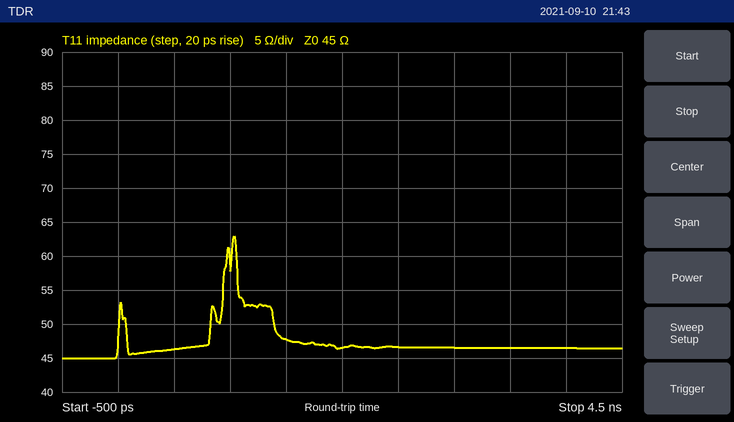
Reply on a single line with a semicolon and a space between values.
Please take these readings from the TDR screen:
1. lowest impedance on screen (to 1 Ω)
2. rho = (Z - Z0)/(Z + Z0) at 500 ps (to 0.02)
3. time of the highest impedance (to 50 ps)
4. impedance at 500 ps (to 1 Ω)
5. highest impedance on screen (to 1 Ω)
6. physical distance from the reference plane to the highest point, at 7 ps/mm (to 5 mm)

45 Ω; +0.02; 1.05 ns; 46 Ω; 63 Ω; 75 mm
